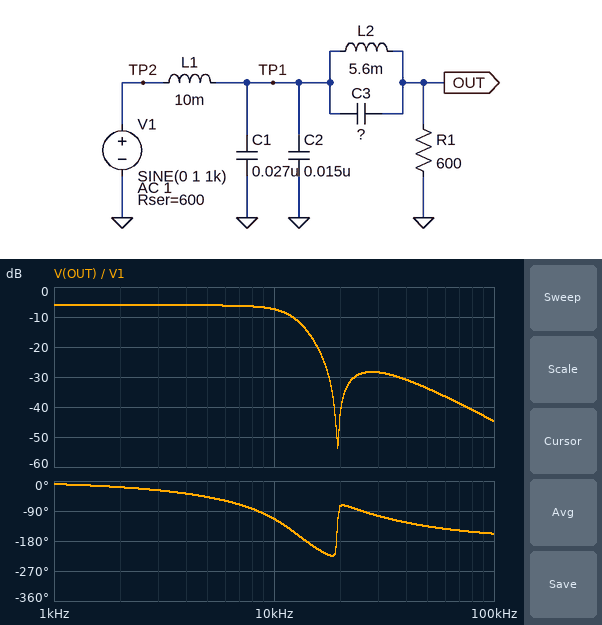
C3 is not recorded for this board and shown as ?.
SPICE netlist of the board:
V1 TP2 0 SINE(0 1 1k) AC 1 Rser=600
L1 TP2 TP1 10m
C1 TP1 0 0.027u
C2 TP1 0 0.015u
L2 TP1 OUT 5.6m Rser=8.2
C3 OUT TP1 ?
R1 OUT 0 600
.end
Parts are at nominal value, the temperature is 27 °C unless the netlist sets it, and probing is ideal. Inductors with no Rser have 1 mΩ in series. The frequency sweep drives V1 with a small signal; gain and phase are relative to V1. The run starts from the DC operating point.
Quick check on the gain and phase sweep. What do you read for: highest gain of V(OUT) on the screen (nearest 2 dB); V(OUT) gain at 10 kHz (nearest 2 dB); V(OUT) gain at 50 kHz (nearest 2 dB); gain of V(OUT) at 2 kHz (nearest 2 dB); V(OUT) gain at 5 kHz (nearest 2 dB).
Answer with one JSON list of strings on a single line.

["-6 dB", "-8 dB", "-34 dB", "-6 dB", "-6 dB"]
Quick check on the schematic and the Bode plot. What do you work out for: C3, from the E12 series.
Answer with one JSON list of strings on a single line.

["12 nF"]
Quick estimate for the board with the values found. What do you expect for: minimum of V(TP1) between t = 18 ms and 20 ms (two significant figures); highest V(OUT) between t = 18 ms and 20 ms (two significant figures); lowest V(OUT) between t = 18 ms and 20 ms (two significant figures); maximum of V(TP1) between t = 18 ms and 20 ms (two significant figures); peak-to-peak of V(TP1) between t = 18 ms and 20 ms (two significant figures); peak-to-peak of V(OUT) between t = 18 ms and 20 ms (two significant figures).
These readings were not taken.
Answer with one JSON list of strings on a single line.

["-500 mV", "500 mV", "-500 mV", "500 mV", "1.0 V", "990 mV"]
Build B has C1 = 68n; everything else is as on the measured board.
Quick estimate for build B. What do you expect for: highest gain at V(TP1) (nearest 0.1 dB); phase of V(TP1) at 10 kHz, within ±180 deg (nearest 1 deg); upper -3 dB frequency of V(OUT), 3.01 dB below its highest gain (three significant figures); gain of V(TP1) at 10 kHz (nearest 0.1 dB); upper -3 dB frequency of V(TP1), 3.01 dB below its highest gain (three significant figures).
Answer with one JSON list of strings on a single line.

["-6.0 dB", "-110 deg", "7.26 kHz", "-10.9 dB", "8.30 kHz"]
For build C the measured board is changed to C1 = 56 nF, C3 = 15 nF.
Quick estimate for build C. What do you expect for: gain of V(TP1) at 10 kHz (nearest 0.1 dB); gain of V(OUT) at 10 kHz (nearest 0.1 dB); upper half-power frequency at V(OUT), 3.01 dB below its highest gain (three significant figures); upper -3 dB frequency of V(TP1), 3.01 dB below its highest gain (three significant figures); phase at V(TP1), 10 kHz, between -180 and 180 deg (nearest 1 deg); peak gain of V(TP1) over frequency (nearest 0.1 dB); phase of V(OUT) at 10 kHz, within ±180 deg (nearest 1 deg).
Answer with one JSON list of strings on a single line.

["-9.2 dB", "-11.8 dB", "8.19 kHz", "9.78 kHz", "-105 deg", "-6.0 dB", "-145 deg"]
